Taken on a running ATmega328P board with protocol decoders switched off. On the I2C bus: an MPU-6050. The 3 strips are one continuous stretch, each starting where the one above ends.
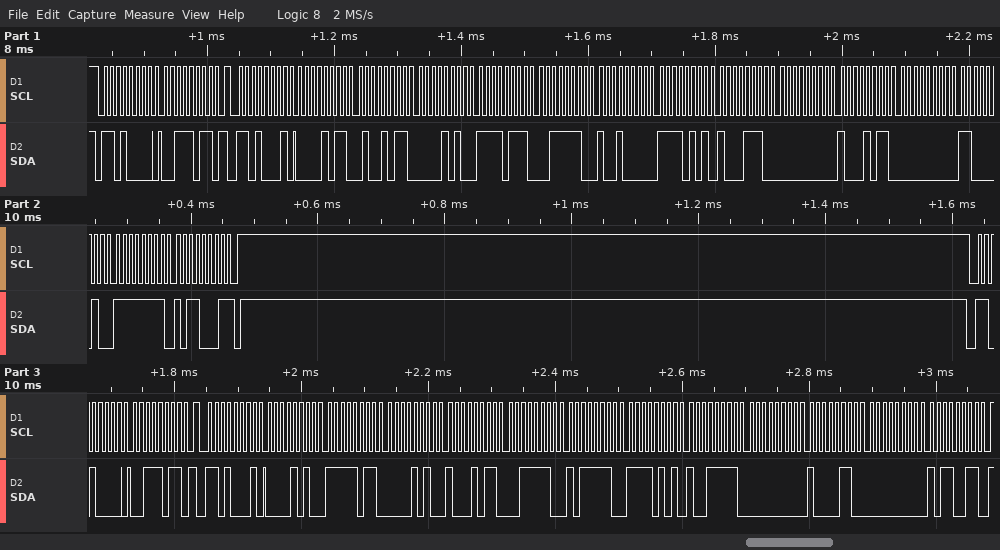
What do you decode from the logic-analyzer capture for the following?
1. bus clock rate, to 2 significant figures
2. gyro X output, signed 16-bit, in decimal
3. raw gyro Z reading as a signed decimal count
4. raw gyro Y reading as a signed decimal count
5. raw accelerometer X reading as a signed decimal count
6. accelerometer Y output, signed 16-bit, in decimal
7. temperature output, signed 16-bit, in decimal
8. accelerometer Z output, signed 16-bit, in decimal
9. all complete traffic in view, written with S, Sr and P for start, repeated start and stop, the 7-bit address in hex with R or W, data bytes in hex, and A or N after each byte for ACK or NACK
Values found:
100 kHz
139
-79
194
2891
2807
-2674
16016
S 68W A 3B A Sr 68R A 0B A 4B A 0A A F7 A 3E A 90 A F5 A 8E A 00 A 8B A 00 A C2 A FF A B1 N P S 68W A 3B A Sr 68R A 0A A FB A 0A A 8B A 3E A BE A F5 A 9F A 00 A 86 A 00 A B3 A
